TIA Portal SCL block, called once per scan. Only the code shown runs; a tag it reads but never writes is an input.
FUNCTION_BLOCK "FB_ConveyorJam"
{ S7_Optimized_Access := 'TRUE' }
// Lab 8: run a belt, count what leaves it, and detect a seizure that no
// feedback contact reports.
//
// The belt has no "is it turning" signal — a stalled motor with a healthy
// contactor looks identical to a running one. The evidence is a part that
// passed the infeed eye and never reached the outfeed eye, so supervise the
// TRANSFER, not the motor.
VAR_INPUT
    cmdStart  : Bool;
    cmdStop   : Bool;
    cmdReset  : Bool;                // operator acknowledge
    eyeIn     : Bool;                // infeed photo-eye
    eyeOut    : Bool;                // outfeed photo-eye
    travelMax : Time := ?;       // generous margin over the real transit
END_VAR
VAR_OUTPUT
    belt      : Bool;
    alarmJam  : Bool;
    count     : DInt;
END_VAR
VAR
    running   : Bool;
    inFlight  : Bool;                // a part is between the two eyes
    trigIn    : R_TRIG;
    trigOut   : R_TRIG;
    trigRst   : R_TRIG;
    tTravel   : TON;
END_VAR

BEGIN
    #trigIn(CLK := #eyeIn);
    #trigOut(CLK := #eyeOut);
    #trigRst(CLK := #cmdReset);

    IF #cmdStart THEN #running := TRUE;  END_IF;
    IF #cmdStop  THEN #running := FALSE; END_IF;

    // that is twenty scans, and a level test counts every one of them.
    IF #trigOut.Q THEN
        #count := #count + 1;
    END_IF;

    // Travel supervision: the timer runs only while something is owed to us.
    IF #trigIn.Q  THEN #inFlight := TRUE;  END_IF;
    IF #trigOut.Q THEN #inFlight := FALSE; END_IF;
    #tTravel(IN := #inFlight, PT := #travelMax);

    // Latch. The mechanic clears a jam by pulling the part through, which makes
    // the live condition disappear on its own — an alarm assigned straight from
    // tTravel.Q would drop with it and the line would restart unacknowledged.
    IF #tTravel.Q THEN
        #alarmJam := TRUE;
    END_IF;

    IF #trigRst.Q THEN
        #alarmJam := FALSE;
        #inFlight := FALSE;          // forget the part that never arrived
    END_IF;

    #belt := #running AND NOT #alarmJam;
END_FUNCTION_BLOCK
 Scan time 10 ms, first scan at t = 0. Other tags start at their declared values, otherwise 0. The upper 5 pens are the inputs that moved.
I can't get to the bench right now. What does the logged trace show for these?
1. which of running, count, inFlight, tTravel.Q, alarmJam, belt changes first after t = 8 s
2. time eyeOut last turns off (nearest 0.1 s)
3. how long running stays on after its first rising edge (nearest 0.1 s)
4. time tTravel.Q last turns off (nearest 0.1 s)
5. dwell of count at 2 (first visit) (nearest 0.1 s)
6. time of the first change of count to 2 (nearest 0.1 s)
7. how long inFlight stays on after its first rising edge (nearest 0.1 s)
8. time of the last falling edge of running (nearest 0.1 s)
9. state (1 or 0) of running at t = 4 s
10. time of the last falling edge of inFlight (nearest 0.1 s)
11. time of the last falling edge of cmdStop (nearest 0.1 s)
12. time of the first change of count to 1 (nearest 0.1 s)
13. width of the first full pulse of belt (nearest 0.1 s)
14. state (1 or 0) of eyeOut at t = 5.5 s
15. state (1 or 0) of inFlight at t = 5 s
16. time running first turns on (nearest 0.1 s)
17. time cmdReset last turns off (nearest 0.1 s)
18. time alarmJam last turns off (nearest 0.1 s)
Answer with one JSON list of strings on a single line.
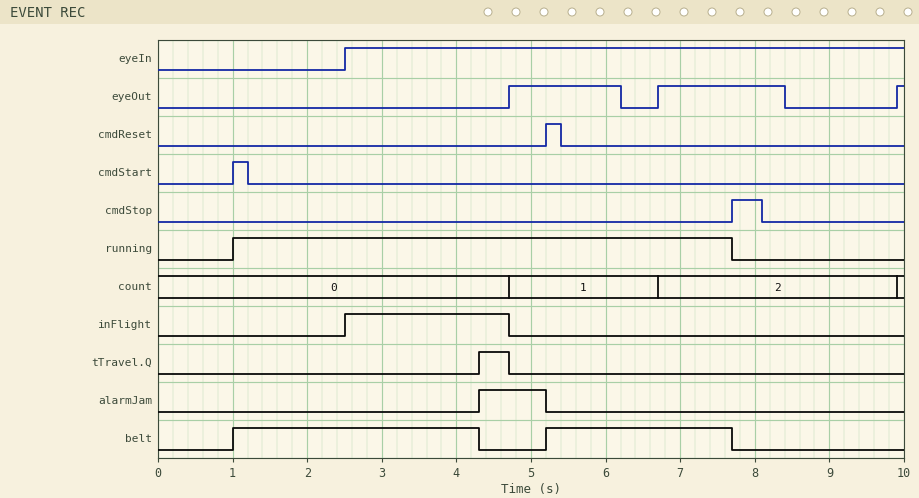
["count", "8.4 s", "6.7 s", "4.7 s", "3.2 s", "6.7 s", "2.2 s", "7.7 s", "1", "4.7 s", "8.1 s", "4.7 s", "3.3 s", "1", "0", "1.0 s", "5.4 s", "5.2 s"]
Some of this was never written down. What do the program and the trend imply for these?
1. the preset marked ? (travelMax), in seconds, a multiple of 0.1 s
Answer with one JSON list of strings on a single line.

["1.8 s"]
